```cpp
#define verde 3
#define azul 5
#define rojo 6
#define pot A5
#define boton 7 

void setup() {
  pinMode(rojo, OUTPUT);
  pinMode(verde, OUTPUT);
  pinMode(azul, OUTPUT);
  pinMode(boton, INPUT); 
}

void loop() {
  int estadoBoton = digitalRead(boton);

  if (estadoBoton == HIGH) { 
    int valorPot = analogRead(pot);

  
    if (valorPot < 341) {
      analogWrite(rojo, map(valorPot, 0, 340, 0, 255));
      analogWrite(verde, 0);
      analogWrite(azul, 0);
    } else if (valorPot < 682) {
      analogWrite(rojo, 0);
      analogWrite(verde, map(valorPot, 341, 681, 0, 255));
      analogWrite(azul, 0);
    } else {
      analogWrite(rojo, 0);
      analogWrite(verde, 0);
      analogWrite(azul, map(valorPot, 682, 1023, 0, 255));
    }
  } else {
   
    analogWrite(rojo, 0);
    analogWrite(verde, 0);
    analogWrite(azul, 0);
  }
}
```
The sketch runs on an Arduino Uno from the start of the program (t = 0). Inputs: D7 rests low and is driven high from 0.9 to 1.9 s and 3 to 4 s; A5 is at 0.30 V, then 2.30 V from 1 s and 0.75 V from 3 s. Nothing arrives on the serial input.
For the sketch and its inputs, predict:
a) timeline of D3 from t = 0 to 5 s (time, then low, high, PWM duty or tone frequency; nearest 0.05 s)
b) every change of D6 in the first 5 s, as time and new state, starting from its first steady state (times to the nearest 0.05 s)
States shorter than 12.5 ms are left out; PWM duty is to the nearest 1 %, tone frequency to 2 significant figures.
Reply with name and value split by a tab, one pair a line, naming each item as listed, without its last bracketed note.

timeline of D3 from t = 0 to 5 s	0 s low; 1 s PWM 38 %; 1.9 s low
every change of D6 in the first 5 s, as time and new state, starting from its first steady state	0 s low; 0.9 s PWM 18 %; 1 s low; 3 s PWM 45 %; 4 s low
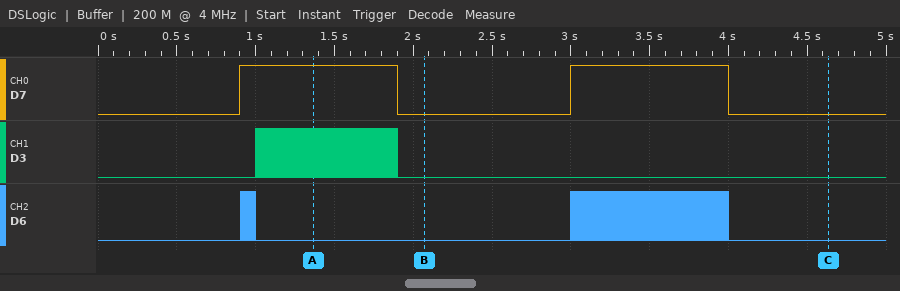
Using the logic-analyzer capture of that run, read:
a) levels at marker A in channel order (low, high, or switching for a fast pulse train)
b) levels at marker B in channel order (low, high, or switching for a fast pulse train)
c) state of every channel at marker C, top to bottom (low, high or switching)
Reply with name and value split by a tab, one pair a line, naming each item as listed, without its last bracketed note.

levels at marker A in channel order	D7 high, D3 switching, D6 low
levels at marker B in channel order	D7 low, D3 low, D6 low
state of every channel at marker C, top to bottom	D7 low, D3 low, D6 low
